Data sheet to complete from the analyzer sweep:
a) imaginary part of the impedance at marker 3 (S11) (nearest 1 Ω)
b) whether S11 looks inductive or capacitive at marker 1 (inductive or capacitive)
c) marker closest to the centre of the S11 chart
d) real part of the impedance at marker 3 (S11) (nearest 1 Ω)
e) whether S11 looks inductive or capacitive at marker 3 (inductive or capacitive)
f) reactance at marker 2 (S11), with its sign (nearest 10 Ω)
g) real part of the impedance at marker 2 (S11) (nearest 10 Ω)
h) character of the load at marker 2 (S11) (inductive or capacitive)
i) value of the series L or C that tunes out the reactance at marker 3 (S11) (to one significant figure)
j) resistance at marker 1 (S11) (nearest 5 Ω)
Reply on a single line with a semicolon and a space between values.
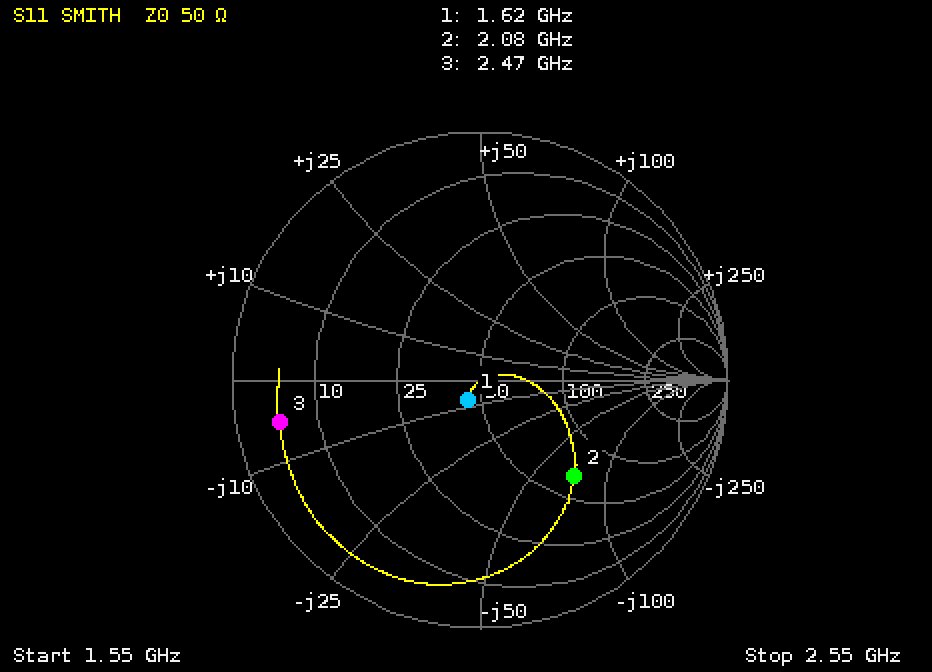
-5 Ω; capacitive; marker 1; 5 Ω; capacitive; -70 Ω; 70 Ω; capacitive; 300 pH; 45 Ω
